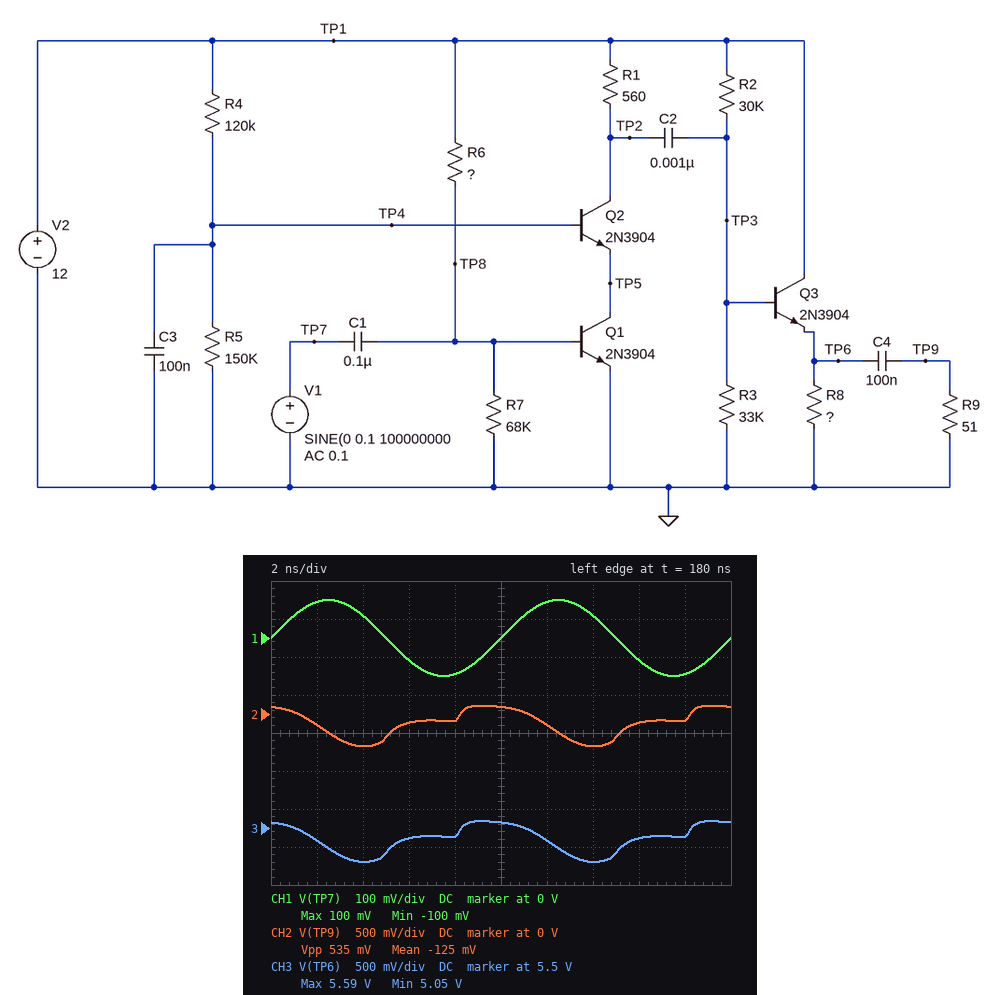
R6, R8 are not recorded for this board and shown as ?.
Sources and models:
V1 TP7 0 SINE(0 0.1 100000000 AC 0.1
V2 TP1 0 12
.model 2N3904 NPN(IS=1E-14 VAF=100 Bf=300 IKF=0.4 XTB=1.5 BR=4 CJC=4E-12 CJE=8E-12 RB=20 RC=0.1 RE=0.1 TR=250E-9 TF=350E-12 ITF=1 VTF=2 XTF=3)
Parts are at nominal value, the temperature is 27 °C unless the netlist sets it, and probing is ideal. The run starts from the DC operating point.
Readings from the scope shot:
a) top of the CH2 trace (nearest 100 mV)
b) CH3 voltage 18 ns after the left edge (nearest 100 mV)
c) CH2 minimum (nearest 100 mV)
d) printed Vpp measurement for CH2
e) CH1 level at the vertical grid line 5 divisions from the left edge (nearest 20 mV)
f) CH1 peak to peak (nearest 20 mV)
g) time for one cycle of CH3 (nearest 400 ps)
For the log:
100 mV
5.4 V
-400 mV
535 mV
0 V
200 mV
10.0 ns
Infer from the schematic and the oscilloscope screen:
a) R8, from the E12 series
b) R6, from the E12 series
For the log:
2.2 kΩ
470 kΩ
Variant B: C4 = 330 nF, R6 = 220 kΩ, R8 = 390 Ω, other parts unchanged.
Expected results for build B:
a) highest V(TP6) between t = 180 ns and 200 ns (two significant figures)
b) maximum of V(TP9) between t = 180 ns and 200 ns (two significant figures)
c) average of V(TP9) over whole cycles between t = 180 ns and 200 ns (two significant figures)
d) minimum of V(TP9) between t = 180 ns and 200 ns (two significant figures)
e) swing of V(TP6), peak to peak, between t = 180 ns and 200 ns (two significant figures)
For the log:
4.4 V
-510 mV
-570 mV
-620 mV
110 mV
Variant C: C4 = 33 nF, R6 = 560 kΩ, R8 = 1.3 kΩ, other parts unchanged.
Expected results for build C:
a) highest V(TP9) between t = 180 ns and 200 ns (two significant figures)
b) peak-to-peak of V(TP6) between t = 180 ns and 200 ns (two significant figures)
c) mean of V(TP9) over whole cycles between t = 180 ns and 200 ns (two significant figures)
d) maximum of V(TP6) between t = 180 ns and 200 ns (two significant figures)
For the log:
4.7 mV
500 mV
-200 mV
5.4 V
